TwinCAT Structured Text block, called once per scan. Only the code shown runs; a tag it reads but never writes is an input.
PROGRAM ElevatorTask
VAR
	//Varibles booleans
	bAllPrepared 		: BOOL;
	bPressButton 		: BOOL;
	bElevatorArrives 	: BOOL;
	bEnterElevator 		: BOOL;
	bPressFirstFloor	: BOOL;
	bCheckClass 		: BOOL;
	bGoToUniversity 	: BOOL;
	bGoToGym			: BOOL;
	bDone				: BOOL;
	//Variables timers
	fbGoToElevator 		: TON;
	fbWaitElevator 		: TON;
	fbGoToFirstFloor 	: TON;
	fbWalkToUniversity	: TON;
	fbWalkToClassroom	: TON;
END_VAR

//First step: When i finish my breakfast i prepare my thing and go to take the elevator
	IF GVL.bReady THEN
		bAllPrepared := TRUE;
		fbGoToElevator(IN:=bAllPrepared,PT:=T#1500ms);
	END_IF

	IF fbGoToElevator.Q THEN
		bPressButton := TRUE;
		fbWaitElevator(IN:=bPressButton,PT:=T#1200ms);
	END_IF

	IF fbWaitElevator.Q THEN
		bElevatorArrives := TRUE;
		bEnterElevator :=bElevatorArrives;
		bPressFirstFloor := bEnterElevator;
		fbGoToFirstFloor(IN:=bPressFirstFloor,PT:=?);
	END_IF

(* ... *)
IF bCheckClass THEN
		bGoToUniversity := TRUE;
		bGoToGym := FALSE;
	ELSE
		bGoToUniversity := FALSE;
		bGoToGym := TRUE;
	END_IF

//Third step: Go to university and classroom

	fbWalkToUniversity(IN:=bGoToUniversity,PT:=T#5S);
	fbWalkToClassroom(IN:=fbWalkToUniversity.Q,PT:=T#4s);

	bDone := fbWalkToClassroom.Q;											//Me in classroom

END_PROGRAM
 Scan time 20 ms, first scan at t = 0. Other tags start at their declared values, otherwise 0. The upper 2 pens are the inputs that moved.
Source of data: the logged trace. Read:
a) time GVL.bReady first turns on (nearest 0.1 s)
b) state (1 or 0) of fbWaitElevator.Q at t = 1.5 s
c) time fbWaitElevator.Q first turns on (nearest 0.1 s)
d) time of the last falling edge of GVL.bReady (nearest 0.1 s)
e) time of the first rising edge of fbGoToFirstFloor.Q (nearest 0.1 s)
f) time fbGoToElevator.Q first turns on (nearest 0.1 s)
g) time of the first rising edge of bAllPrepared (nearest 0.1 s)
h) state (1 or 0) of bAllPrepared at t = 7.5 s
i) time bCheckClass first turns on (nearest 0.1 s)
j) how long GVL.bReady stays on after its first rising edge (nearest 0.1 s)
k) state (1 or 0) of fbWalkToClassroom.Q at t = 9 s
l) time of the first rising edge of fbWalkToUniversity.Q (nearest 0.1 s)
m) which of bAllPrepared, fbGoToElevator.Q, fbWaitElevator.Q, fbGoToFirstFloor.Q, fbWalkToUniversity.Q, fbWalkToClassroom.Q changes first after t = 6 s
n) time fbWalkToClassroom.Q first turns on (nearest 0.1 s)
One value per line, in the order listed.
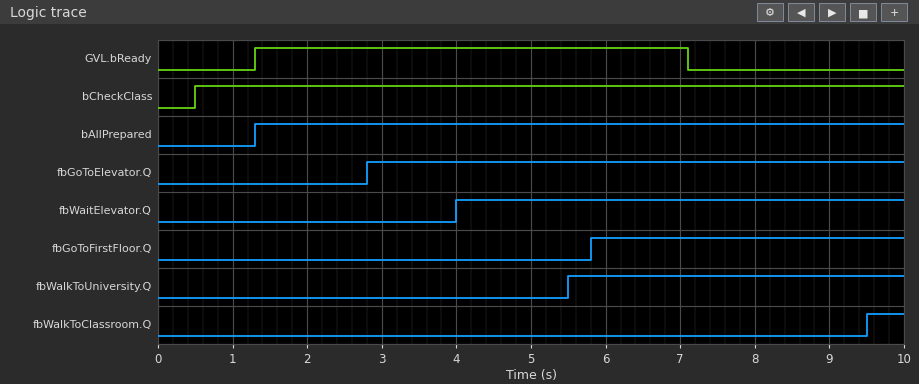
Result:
1.3 s
0
4.0 s
7.1 s
5.8 s
2.8 s
1.3 s
1
0.5 s
5.8 s
0
5.5 s
fbWalkToClassroom.Q
9.5 s
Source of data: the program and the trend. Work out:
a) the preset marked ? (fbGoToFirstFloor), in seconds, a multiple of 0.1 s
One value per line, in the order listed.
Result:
1.8 s
